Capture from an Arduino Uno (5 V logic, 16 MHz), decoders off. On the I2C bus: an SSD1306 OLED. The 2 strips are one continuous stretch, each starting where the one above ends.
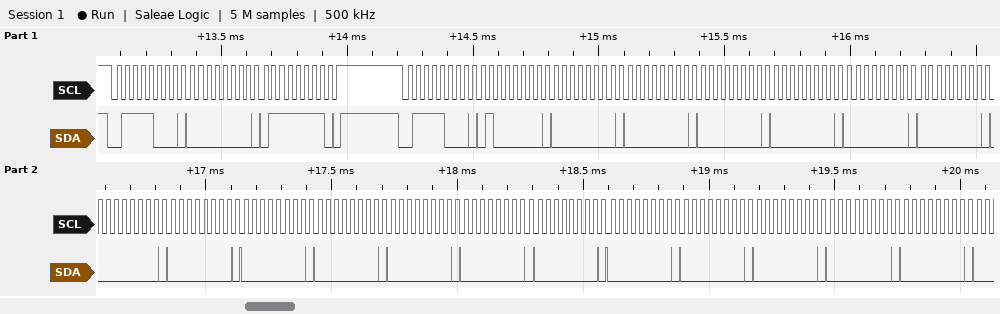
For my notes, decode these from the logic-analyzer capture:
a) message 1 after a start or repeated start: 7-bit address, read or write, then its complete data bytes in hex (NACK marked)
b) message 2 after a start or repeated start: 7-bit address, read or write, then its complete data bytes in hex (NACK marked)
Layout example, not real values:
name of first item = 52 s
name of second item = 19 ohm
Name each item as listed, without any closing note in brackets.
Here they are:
message 1 after a start or repeated start: 7-bit address, read or write, then its complete data bytes in hex = 0x3C write: 00 7F
message 2 after a start or repeated start: 7-bit address, read or write, then its complete data bytes in hex = 0x3C write: 40 00 00 00 00 00 00 00 00 00 00 00 00 00 00 00 00 00 00
